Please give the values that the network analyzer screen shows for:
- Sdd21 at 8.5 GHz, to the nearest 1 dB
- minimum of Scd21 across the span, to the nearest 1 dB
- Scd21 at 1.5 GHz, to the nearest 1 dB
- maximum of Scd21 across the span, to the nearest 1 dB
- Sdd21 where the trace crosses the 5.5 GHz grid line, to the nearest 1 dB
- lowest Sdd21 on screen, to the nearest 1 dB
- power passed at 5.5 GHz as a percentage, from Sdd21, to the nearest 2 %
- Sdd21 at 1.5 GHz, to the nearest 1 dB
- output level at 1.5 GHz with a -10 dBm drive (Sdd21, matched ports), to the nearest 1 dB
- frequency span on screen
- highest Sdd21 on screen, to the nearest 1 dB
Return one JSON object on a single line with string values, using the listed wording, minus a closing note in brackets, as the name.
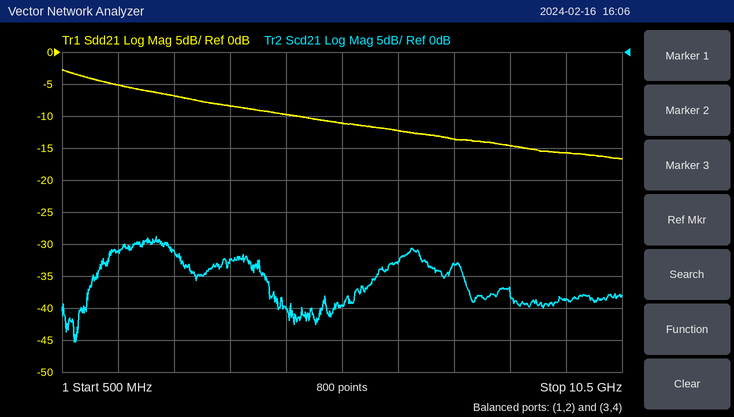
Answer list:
{"Sdd21 at 8.5 GHz, to the nearest 1 dB": "-15 dB", "minimum of Scd21 across the span, to the nearest 1 dB": "-45 dB", "Scd21 at 1.5 GHz, to the nearest 1 dB": "-31 dB", "maximum of Scd21 across the span, to the nearest 1 dB": "-29 dB", "Sdd21 where the trace crosses the 5.5 GHz grid line, to the nearest 1 dB": "-11 dB", "lowest Sdd21 on screen, to the nearest 1 dB": "-17 dB", "power passed at 5.5 GHz as a percentage, from Sdd21, to the nearest 2 %": "8 %", "Sdd21 at 1.5 GHz, to the nearest 1 dB": "-5 dB", "output level at 1.5 GHz with a -10 dBm drive (Sdd21, matched ports), to the nearest 1 dB": "-15 dBm", "frequency span on screen": "10 GHz", "highest Sdd21 on screen, to the nearest 1 dB": "-3 dB"}
